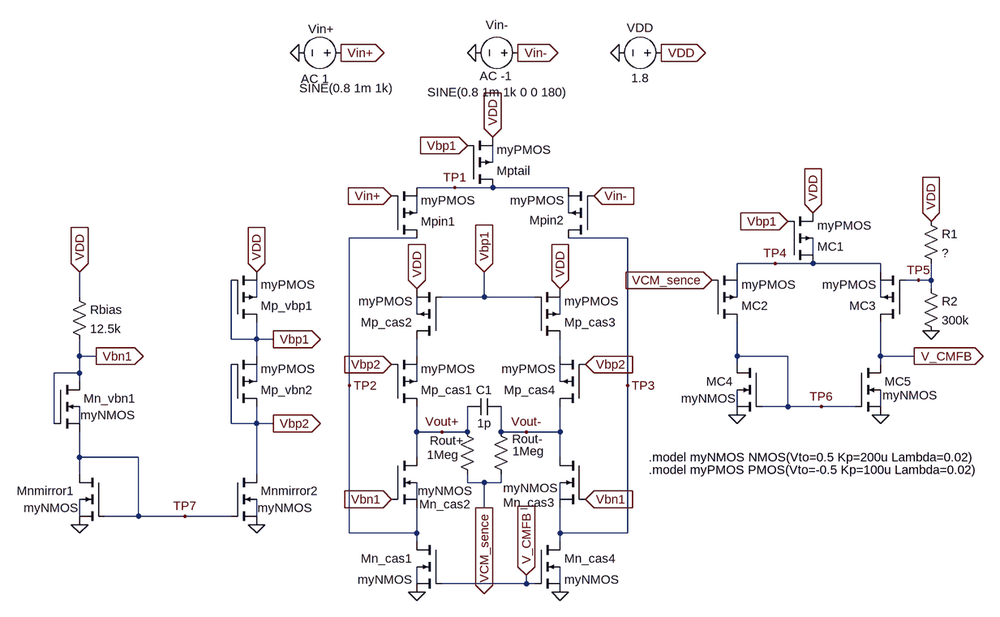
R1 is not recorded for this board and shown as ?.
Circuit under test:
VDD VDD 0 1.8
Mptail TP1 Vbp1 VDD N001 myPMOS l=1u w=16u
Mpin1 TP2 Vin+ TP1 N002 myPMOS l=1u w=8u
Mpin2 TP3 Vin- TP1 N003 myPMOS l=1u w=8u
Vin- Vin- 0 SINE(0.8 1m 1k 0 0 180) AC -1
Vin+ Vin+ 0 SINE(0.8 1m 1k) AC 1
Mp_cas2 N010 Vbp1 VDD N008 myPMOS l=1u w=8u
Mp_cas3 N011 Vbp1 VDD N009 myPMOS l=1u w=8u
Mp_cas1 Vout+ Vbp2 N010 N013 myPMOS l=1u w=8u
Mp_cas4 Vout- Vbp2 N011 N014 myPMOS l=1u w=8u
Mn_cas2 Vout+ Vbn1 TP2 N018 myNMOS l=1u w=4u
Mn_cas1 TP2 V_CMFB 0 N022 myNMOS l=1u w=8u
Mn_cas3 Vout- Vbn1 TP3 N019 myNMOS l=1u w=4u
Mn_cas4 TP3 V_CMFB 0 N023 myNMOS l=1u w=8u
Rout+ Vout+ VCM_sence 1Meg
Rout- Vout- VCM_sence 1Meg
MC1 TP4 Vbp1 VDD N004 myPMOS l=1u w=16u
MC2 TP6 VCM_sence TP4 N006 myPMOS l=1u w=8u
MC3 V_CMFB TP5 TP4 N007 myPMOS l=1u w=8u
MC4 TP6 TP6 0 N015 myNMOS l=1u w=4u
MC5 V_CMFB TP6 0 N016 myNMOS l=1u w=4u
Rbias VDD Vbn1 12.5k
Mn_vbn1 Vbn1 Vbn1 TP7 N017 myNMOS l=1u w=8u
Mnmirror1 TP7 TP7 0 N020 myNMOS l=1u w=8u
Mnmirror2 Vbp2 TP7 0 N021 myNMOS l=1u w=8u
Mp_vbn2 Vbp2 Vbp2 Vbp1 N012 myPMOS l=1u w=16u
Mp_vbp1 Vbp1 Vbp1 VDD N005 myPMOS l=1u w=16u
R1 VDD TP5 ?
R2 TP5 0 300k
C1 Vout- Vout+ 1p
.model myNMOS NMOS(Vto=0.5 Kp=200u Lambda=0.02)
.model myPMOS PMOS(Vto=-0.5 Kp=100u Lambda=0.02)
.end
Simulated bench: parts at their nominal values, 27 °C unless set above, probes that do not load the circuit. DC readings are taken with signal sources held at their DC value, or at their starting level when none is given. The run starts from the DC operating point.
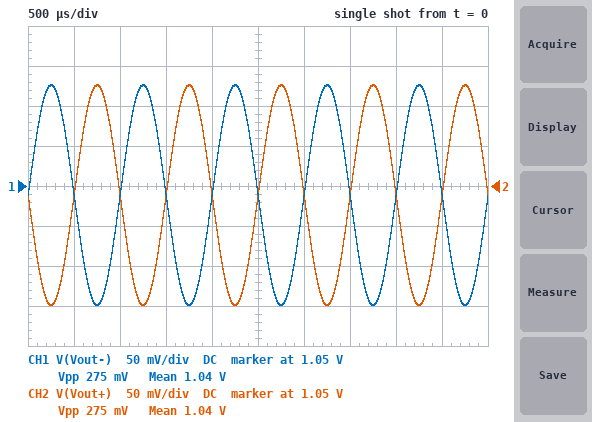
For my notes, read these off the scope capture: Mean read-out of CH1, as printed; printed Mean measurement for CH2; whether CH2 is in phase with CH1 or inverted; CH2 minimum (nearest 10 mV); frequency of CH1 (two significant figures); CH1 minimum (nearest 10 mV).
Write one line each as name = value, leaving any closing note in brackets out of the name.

Mean read-out of CH1, as printed = 1.04 V
printed Mean measurement for CH2 = 1.04 V
whether CH2 is in phase with CH1 or inverted = inverted
CH2 minimum = 900 mV
frequency of CH1 = 1.0 kHz
CH1 minimum = 900 mV
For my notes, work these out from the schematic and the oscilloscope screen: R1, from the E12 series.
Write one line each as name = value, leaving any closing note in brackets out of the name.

R1, from the E12 series = 220 kΩ
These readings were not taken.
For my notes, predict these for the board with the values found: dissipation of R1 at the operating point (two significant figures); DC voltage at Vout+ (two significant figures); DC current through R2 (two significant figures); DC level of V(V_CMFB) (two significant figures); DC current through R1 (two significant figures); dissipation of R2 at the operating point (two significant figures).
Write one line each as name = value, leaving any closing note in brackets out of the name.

dissipation of R1 at the operating point = 2.6 µW
DC voltage at Vout+ = 1.0 V
DC current through R2 = 3.5 µA
DC level of V(V_CMFB) = 700 mV
DC current through R1 = 3.5 µA
dissipation of R2 at the operating point = 3.6 µW
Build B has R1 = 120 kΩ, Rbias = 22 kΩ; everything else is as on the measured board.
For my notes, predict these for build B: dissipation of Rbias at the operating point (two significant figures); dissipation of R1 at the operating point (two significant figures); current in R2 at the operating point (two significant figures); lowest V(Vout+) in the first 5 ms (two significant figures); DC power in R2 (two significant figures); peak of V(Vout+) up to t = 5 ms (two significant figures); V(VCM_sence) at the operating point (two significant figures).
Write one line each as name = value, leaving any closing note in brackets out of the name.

dissipation of Rbias at the operating point = 10 µW
dissipation of R1 at the operating point = 2.2 µW
current in R2 at the operating point = 4.3 µA
lowest V(Vout+) in the first 5 ms = 1.2 V
DC power in R2 = 5.5 µW
peak of V(Vout+) up to t = 5 ms = 1.4 V
V(VCM_sence) at the operating point = 1.3 V
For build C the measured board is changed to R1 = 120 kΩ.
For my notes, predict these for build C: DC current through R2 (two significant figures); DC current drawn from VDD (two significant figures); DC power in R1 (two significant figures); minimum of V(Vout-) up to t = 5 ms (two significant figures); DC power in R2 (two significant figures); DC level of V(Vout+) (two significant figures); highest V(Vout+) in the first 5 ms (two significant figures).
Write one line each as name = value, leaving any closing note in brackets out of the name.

DC current through R2 = 4.3 µA
DC current drawn from VDD = 130 µA
DC power in R1 = 2.2 µW
minimum of V(Vout-) up to t = 5 ms = 1.2 V
DC power in R2 = 5.5 µW
DC level of V(Vout+) = 1.3 V
highest V(Vout+) in the first 5 ms = 1.4 V
